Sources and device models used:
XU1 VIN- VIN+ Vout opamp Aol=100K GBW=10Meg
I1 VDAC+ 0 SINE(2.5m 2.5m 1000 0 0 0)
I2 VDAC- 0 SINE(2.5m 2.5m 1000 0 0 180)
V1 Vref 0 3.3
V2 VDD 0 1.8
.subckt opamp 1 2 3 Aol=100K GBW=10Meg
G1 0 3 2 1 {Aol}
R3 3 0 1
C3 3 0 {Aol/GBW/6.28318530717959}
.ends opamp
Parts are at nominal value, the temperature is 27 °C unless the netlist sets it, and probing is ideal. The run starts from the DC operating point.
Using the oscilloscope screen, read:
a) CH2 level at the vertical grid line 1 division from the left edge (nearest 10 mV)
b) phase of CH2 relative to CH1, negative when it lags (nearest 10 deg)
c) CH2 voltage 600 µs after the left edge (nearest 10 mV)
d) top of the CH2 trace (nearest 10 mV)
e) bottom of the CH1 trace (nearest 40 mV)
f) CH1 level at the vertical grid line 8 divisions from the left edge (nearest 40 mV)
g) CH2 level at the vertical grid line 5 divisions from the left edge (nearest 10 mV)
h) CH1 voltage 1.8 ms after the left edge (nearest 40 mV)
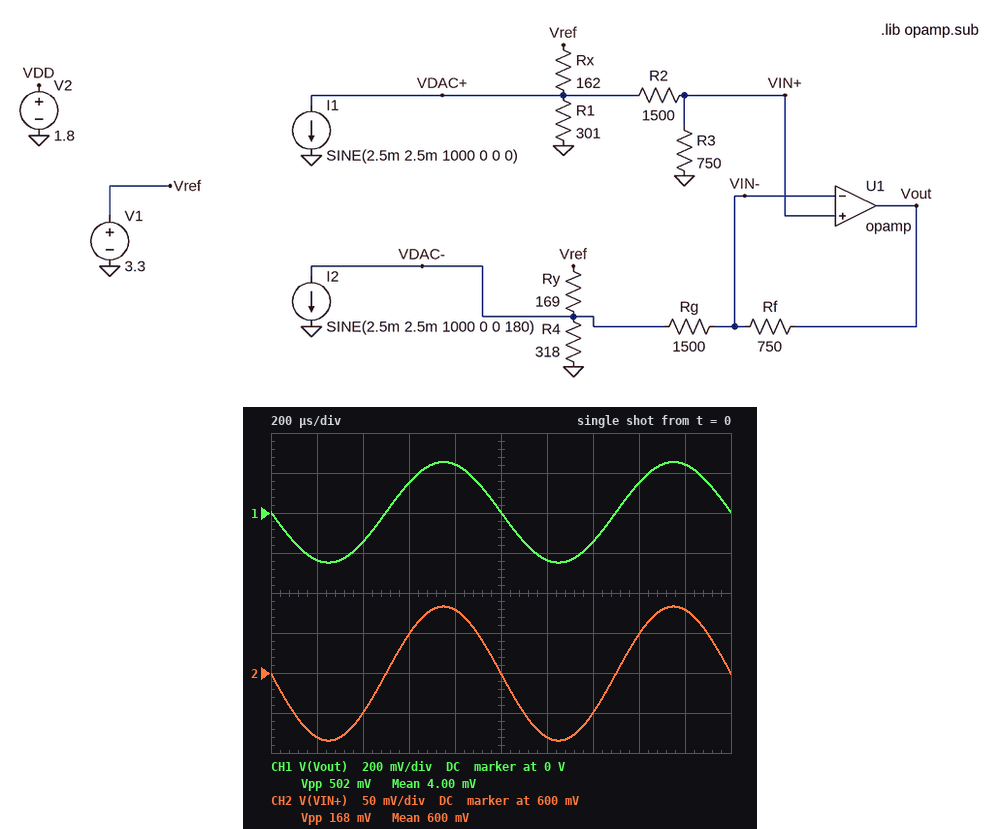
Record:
520 mV
0 deg
650 mV
680 mV
-240 mV
160 mV
600 mV
240 mV
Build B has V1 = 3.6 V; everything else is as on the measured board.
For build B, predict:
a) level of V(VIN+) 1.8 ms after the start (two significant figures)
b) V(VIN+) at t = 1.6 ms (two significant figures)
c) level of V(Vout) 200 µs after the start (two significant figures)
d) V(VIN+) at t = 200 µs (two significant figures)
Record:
740 mV
710 mV
-240 mV
580 mV
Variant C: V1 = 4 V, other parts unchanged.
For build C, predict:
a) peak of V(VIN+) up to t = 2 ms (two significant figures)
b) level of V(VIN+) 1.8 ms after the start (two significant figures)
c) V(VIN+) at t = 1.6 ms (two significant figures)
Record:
830 mV
820 mV
790 mV
